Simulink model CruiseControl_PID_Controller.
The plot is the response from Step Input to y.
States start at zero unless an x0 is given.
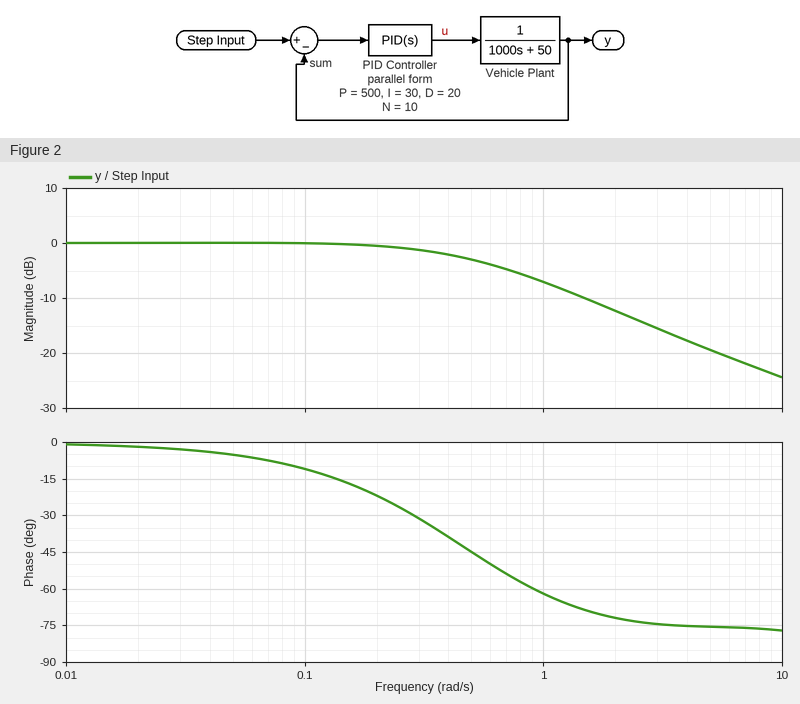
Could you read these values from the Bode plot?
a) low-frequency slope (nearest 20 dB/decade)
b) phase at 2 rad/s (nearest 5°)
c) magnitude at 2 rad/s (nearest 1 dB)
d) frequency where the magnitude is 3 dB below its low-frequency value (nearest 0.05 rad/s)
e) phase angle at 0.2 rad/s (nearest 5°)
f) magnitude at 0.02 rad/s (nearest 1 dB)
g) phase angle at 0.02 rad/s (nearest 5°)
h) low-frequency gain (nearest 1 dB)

0 dB/decade
-70°
-12 dB
0.50 rad/s
-20°
0 dB
0°
0 dB
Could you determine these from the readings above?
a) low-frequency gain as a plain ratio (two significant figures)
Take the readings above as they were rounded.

1.0
